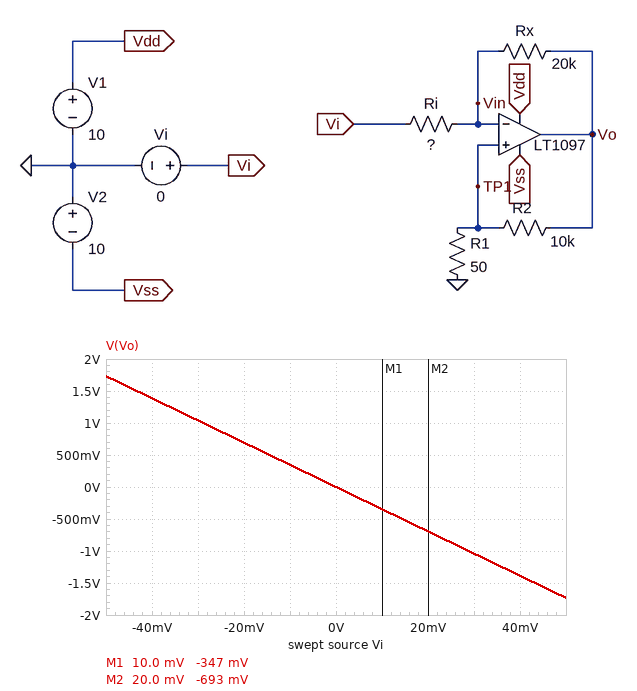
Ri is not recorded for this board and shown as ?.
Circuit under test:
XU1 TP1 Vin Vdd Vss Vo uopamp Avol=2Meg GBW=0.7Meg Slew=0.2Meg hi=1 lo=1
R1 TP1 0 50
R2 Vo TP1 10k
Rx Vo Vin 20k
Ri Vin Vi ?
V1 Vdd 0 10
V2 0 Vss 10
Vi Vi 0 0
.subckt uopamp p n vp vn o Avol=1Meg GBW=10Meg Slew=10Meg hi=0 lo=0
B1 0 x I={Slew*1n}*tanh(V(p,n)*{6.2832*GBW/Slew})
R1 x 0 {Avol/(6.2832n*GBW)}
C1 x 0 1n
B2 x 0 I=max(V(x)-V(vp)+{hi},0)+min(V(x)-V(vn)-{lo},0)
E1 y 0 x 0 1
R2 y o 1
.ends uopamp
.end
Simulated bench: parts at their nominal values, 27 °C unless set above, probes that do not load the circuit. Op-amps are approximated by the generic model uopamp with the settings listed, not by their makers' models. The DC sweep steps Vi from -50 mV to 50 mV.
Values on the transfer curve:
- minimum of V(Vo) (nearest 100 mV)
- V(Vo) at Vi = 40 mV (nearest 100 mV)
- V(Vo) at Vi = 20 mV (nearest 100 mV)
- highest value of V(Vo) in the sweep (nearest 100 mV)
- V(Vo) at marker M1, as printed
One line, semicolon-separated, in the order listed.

-1.7 V; -1.4 V; -700 mV; 1.7 V; -347 mV
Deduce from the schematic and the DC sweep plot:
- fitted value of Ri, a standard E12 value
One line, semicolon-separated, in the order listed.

680 Ω
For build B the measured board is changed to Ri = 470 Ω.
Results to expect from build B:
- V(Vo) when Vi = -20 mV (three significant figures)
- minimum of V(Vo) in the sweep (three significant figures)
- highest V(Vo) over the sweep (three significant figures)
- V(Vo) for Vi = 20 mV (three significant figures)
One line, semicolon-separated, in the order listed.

1.09 V; -2.72 V; 2.72 V; -1.09 V
